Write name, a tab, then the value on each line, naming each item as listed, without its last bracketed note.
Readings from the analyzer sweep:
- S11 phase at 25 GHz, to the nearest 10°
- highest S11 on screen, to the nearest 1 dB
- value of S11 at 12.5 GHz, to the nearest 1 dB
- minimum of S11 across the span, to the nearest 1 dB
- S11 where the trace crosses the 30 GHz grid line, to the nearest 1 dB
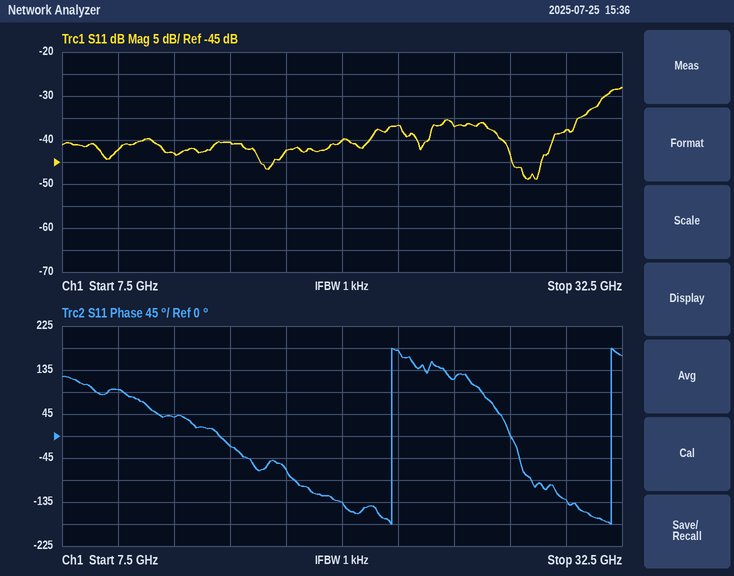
S11 phase at 25 GHz, to the nearest 10°	120°
highest S11 on screen, to the nearest 1 dB	-28 dB
value of S11 at 12.5 GHz, to the nearest 1 dB	-43 dB
minimum of S11 across the span, to the nearest 1 dB	-49 dB
S11 where the trace crosses the 30 GHz grid line, to the nearest 1 dB	-38 dB
